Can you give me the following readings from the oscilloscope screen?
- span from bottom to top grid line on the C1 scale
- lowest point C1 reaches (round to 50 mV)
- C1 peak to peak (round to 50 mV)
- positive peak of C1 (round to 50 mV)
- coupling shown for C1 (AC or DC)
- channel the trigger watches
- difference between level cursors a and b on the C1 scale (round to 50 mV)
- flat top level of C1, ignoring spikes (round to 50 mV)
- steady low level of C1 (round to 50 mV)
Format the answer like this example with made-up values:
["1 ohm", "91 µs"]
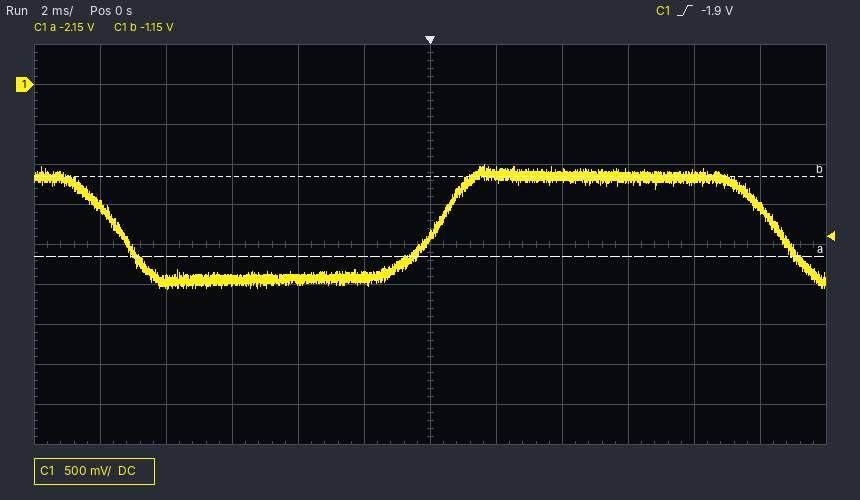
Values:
["5 V", "-2.55 V", "1.55 V", "-1.00 V", "DC", "C1", "1.00 V", "-1.15 V", "-2.45 V"]
